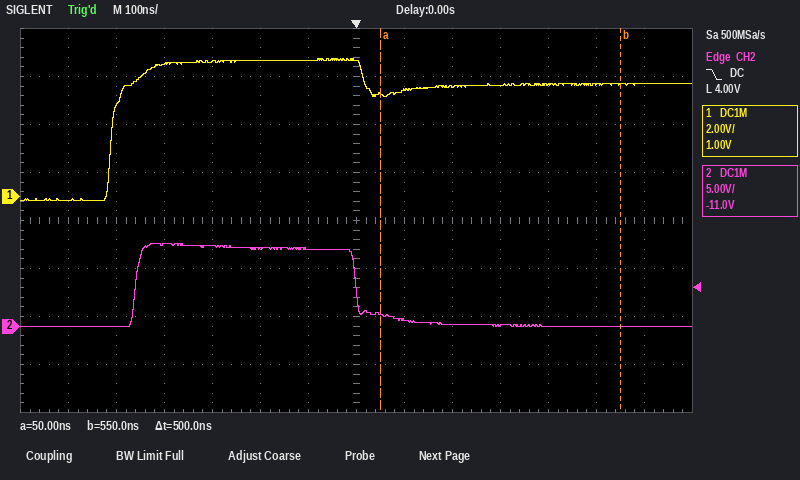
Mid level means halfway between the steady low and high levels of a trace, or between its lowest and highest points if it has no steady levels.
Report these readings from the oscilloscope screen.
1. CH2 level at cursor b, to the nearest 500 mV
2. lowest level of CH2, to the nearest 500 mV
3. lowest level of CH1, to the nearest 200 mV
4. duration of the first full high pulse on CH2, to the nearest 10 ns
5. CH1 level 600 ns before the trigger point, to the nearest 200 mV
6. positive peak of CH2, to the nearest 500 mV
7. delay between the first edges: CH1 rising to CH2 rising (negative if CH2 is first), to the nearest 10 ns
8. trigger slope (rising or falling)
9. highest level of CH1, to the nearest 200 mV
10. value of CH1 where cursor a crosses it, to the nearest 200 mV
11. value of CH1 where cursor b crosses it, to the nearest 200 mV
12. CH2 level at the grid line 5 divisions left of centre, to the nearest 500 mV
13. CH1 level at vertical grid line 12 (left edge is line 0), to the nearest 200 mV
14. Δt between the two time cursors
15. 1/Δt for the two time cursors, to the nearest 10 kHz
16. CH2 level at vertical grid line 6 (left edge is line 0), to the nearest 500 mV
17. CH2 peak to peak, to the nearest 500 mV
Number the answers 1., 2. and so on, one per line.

1. 0.0 V
2. 0.0 V
3. -200 mV
4. 460 ns
5. -200 mV
6. 8.5 V
7. +50 ns
8. falling
9. 5.8 V
10. 4.2 V
11. 4.6 V
12. 0.0 V
13. 4.6 V
14. 500 ns
15. 2.00 MHz
16. 8.0 V
17. 8.5 V
